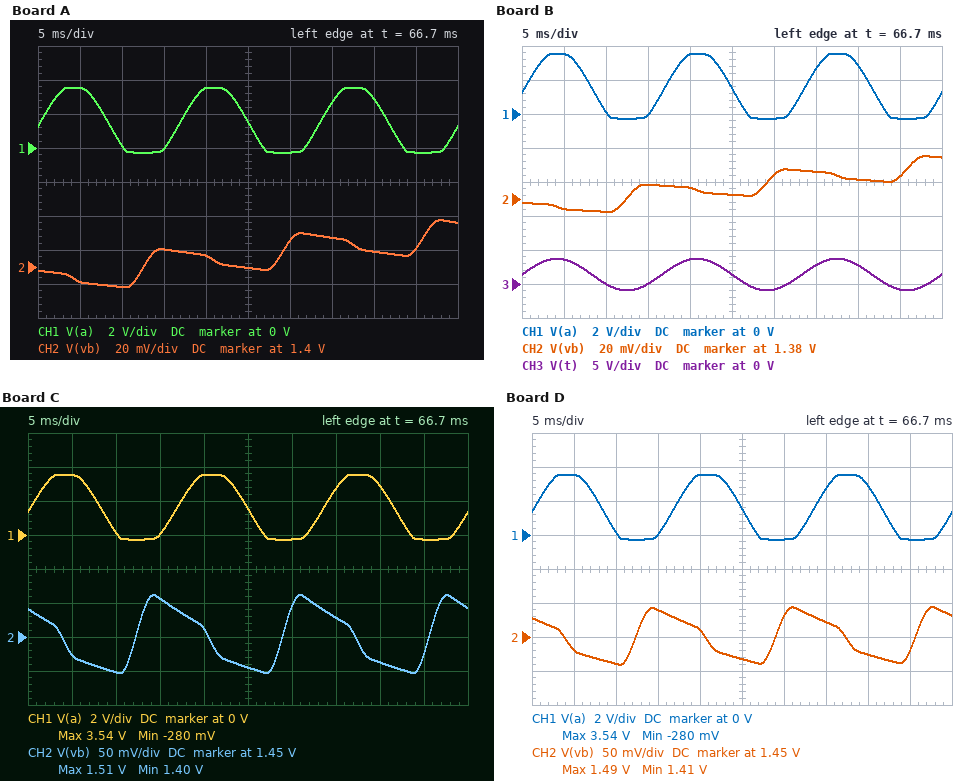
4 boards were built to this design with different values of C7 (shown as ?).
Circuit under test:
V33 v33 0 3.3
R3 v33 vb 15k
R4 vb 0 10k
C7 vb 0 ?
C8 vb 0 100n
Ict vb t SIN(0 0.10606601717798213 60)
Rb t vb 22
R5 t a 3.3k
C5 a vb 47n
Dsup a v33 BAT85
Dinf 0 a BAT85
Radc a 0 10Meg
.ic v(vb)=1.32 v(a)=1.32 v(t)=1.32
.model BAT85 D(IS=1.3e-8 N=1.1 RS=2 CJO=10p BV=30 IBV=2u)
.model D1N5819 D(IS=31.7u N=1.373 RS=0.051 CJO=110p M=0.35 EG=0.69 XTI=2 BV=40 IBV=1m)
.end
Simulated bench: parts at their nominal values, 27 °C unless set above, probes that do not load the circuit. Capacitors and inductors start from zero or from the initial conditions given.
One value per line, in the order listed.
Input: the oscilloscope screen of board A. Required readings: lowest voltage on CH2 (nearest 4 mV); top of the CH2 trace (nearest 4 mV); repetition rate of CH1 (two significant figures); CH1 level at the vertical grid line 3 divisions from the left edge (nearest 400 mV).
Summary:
1.388 V
1.428 V
60 Hz
0 V
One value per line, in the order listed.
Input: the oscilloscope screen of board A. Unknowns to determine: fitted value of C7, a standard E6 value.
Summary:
22 µF
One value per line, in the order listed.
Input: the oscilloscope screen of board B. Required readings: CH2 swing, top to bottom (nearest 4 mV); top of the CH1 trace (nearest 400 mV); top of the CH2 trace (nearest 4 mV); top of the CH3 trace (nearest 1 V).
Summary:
32 mV
3.6 V
1.404 V
4 V
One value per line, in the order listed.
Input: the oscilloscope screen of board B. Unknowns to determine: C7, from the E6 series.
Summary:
33 µF
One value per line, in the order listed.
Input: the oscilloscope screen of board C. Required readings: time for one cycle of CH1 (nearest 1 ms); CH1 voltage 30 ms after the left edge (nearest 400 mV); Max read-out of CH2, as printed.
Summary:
17 ms
-400 mV
1.51 V
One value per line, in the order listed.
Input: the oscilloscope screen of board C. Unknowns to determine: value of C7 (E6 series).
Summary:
3.3 µF
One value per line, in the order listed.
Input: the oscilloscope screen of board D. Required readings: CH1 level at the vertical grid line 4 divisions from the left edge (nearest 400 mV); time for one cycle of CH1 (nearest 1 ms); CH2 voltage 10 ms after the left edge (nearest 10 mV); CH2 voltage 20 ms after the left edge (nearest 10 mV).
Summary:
3.6 V
17 ms
1.41 V
1.46 V
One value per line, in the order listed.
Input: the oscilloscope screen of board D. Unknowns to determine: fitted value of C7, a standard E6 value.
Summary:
4.7 µF
